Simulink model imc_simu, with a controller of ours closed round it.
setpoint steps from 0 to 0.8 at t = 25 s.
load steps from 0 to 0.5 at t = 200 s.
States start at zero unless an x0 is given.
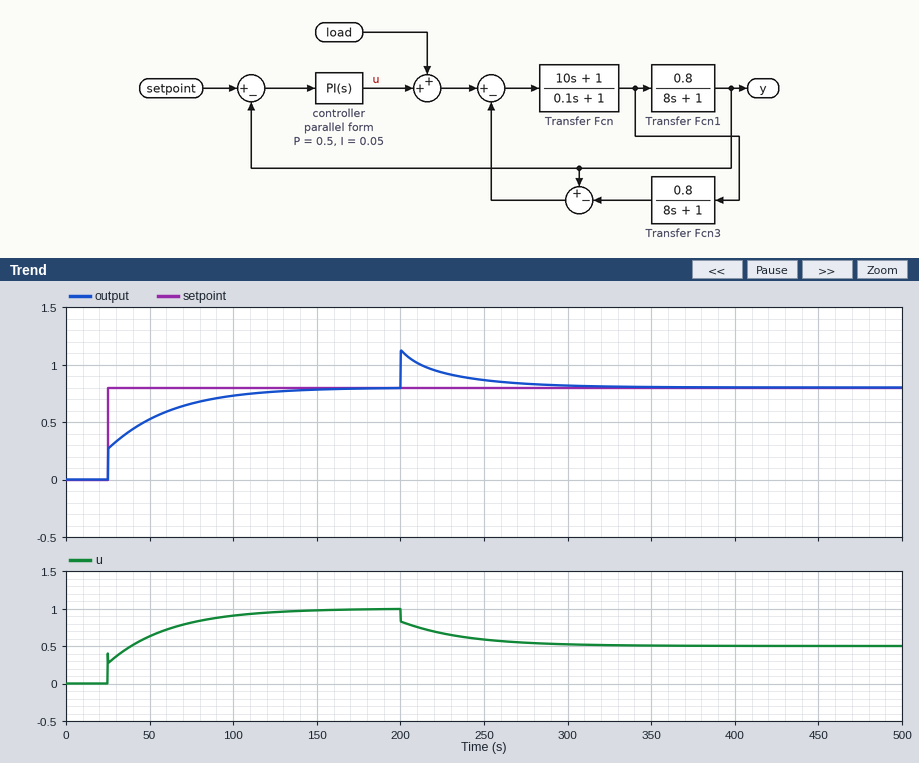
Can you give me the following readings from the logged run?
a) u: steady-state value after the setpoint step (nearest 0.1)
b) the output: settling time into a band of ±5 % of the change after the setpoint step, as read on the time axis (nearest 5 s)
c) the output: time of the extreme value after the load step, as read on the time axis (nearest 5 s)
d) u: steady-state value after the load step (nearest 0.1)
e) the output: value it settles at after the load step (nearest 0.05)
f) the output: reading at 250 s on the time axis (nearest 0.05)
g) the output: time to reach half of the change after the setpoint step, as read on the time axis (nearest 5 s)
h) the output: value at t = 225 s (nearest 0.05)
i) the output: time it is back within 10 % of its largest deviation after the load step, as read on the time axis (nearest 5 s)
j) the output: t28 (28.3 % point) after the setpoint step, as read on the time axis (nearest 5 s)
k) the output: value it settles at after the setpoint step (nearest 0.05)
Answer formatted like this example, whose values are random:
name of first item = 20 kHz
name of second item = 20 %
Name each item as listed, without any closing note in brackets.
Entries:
u: steady-state value after the setpoint step = 1.0
the output: settling time into a band of ±5 % of the change after the setpoint step, as read on the time axis = 120 s
the output: time of the extreme value after the load step, as read on the time axis = 200 s
u: steady-state value after the load step = 0.5
the output: value it settles at after the load step = 0.80
the output: reading at 250 s on the time axis = 0.85
the output: time to reach half of the change after the setpoint step, as read on the time axis = 35 s
the output: value at t = 225 s = 0.95
the output: time it is back within 10 % of its largest deviation after the load step, as read on the time axis = 275 s
the output: t28 (28.3 % point) after the setpoint step, as read on the time axis = 25 s
the output: value it settles at after the setpoint step = 0.80
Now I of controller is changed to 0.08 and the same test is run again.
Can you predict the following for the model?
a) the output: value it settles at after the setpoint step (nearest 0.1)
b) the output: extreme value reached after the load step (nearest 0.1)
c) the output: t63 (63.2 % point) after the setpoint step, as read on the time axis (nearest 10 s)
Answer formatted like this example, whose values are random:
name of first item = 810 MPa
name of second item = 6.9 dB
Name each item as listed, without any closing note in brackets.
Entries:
the output: value it settles at after the setpoint step = 0.8
the output: extreme value reached after the load step = 1.1
the output: t63 (63.2 % point) after the setpoint step, as read on the time axis = 40 s
